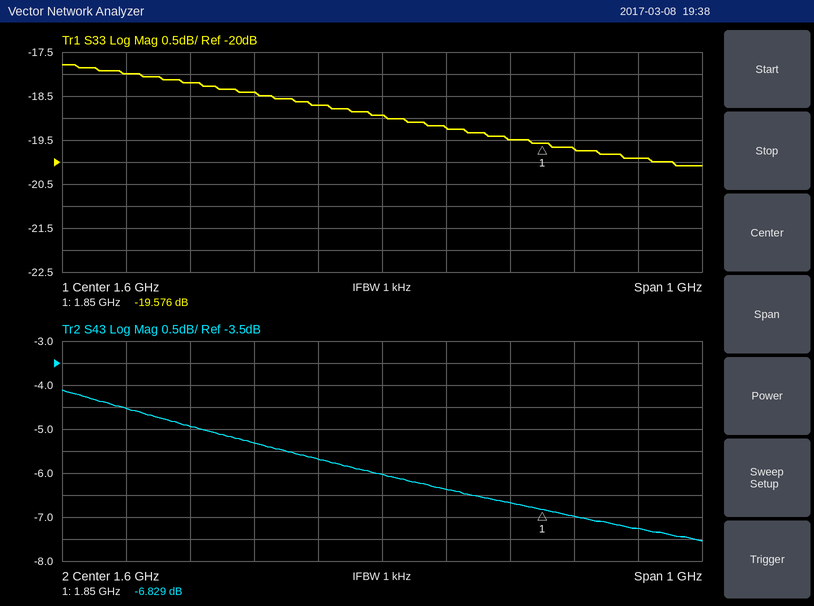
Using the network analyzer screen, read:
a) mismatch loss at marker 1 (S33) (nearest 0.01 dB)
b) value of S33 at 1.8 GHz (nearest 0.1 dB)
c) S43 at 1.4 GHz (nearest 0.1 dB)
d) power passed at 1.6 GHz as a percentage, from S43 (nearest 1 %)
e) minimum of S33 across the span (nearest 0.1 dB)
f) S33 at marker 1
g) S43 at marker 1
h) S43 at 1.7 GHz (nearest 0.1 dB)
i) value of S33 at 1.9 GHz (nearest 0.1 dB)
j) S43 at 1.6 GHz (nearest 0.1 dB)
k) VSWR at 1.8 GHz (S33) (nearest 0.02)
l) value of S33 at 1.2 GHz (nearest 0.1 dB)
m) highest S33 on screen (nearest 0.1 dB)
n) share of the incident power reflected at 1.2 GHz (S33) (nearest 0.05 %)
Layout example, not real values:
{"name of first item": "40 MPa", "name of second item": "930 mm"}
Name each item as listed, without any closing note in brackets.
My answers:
{"mismatch loss at marker 1 (S33)": "0.05 dB", "value of S33 at 1.8 GHz": "-19.5 dB", "S43 at 1.4 GHz": "-5.3 dB", "power passed at 1.6 GHz as a percentage, from S43": "25 %", "minimum of S33 across the span": "-20.1 dB", "S33 at marker 1": "-19.576 dB", "S43 at marker 1": "-6.829 dB", "S43 at 1.7 GHz": "-6.4 dB", "value of S33 at 1.9 GHz": "-19.7 dB", "S43 at 1.6 GHz": "-6.0 dB", "VSWR at 1.8 GHz (S33)": "1.24", "value of S33 at 1.2 GHz": "-18.0 dB", "highest S33 on screen": "-17.8 dB", "share of the incident power reflected at 1.2 GHz (S33)": "1.60 %"}
